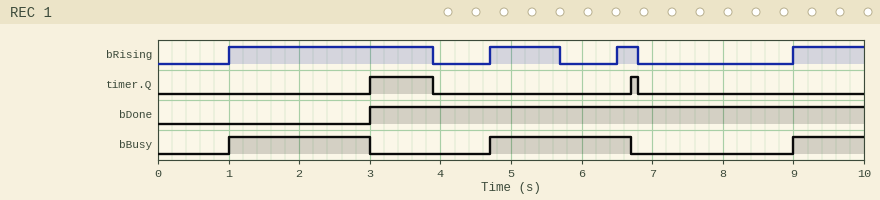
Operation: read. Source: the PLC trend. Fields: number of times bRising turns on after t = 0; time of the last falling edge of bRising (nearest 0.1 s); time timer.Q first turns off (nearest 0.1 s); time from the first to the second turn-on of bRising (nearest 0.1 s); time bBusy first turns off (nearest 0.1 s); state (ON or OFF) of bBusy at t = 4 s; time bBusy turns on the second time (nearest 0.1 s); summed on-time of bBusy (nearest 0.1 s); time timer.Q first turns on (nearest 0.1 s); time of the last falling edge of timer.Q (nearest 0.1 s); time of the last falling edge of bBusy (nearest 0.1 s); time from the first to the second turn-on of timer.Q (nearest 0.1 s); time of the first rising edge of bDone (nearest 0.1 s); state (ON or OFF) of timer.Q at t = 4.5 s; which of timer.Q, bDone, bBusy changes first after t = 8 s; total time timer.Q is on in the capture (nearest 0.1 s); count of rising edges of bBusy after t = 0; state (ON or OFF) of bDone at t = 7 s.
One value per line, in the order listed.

4
6.8 s
3.9 s
3.7 s
3.0 s
OFF
4.7 s
5.0 s
3.0 s
6.8 s
6.7 s
3.7 s
3.0 s
OFF
bBusy
1.0 s
3
ON
